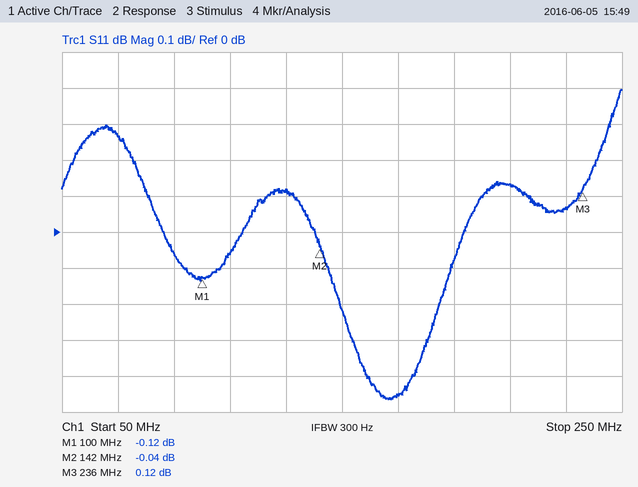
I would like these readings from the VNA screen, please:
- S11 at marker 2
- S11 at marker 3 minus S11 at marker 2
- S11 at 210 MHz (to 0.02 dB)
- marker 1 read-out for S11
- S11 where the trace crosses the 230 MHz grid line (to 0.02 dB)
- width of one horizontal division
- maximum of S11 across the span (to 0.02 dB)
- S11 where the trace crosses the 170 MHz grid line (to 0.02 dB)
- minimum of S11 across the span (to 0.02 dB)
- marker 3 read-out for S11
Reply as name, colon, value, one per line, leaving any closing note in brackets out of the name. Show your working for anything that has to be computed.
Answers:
S11 at marker 2: -0.04 dB
S11 at marker 3 minus S11 at marker 2: 0.12 − (-0.04) = 0.16 dB
S11 at 210 MHz: 0.14 dB
marker 1 read-out for S11: -0.12 dB
S11 where the trace crosses the 230 MHz grid line: 0.06 dB
width of one horizontal division: 20 MHz
maximum of S11 across the span: 0.40 dB
S11 where the trace crosses the 170 MHz grid line: -0.46 dB
minimum of S11 across the span: -0.46 dB
marker 3 read-out for S11: 0.12 dB
